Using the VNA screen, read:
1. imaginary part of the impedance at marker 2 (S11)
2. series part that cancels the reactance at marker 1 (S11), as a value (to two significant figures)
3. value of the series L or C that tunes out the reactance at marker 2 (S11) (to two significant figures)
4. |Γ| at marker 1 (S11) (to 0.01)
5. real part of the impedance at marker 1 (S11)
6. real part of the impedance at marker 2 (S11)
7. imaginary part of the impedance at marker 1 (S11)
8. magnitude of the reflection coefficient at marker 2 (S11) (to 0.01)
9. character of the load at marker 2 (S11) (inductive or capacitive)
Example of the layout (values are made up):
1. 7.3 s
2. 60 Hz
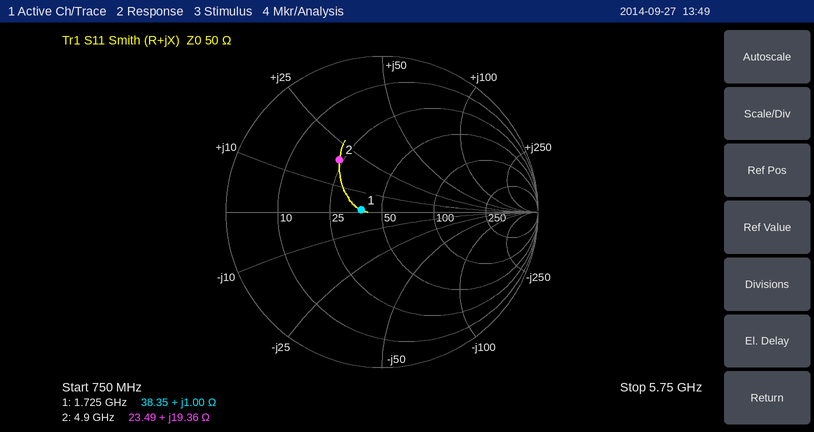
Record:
1. +19.36 Ω
2. 92 pF
3. 1.7 pF
4. 0.13
5. 38.35 Ω
6. 23.49 Ω
7. +1.00 Ω
8. 0.43
9. inductive
